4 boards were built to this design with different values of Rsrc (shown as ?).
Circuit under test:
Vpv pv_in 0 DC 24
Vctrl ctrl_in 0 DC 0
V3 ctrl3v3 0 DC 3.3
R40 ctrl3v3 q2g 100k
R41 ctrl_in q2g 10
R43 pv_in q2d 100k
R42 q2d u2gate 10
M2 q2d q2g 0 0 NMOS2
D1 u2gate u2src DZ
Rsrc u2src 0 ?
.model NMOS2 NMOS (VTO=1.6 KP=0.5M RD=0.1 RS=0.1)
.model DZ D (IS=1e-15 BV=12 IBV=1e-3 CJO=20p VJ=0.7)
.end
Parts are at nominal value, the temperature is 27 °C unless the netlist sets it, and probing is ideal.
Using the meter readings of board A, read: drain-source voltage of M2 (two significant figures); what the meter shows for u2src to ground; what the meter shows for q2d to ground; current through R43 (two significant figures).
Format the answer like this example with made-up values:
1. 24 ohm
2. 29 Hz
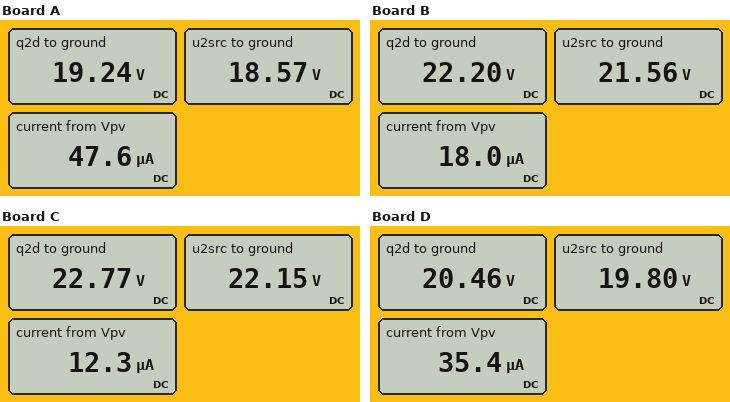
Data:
1. 19 V
2. 18.57 V
3. 19.24 V
4. 48 µA
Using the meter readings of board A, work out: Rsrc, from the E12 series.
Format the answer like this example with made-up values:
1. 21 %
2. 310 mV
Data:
1. 390 kΩ
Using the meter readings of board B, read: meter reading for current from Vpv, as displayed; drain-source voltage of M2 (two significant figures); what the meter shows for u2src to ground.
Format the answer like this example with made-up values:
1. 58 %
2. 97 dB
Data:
1. 18.0 µA
2. 22 V
3. 21.56 V
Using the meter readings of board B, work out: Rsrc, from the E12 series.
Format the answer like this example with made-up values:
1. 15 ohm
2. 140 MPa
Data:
1. 1.2 MΩ
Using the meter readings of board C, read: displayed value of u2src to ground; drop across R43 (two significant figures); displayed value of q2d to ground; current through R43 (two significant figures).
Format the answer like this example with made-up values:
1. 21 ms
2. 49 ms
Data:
1. 22.15 V
2. 1.2 V
3. 22.77 V
4. 12 µA
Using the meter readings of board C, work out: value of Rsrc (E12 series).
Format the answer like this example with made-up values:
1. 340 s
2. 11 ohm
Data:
1. 1.8 MΩ
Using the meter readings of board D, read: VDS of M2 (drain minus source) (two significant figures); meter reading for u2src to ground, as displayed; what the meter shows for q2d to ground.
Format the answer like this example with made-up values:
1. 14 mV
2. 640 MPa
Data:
1. 20 V
2. 19.80 V
3. 20.46 V
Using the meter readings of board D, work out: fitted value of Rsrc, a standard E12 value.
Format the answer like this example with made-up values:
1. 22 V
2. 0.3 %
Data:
1. 560 kΩ
